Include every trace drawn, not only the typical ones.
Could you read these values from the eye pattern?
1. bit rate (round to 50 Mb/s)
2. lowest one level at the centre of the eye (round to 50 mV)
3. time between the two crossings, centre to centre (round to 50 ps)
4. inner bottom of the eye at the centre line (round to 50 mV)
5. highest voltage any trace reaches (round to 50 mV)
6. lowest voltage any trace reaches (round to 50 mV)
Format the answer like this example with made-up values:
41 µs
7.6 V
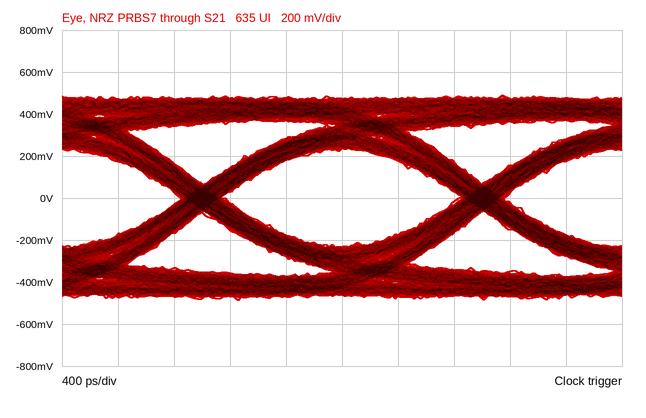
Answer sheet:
500 Mb/s
250 mV
2.00 ns
-250 mV
500 mV
-500 mV
